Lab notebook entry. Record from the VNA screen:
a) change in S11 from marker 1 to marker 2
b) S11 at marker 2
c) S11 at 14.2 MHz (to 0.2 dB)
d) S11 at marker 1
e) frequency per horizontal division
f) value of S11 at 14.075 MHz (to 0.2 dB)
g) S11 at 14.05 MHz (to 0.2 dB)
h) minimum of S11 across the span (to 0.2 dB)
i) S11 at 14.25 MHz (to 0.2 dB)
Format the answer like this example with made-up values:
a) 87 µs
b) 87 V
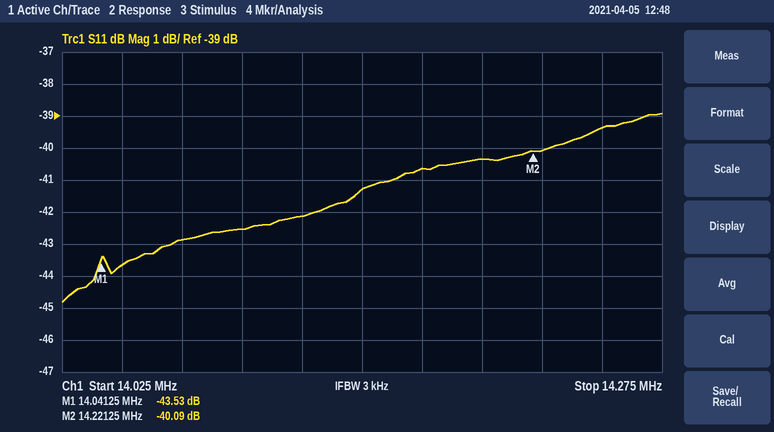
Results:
a) 3.44 dB
b) -40.09 dB
c) -40.4 dB
d) -43.53 dB
e) 25 kHz
f) -42.8 dB
g) -43.6 dB
h) -44.8 dB
i) -39.4 dB
